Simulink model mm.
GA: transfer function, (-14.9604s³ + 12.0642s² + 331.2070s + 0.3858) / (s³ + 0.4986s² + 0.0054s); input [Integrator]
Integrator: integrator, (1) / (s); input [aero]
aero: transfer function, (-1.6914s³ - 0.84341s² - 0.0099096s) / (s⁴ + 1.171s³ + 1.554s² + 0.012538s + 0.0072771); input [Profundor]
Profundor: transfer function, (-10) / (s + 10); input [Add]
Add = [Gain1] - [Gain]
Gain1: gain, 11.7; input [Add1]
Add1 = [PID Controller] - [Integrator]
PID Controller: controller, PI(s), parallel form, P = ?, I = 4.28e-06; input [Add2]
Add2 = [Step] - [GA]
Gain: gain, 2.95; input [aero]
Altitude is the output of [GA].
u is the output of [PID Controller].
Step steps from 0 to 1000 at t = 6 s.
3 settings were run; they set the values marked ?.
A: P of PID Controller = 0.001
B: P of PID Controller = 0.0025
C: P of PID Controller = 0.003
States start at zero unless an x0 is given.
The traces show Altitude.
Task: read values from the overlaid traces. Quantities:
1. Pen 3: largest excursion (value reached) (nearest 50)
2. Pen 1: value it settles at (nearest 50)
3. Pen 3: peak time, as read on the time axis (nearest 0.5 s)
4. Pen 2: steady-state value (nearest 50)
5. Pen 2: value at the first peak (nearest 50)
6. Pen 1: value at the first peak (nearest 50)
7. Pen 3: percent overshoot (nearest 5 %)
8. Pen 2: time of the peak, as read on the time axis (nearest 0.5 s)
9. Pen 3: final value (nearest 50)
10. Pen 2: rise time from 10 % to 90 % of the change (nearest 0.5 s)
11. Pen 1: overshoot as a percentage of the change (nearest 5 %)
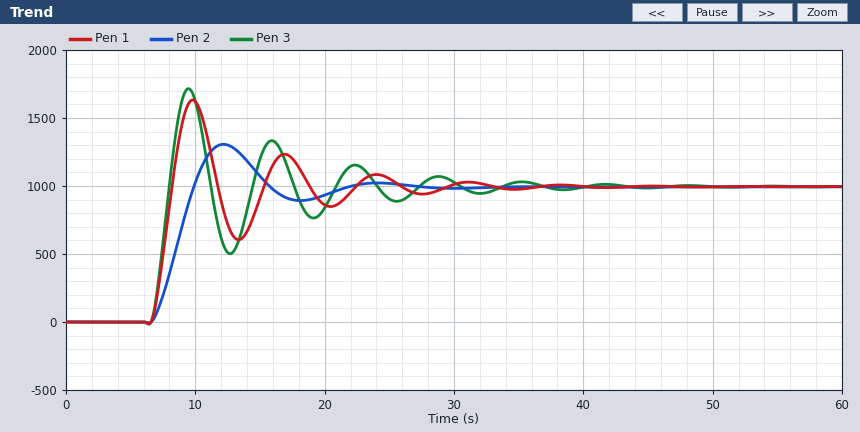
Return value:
1700
1000
9.5 s
1000
1300
1650
70 %
12.0 s
1000
2.5 s
65 %
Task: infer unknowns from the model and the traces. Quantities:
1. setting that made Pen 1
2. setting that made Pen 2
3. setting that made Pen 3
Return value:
B
A
C
